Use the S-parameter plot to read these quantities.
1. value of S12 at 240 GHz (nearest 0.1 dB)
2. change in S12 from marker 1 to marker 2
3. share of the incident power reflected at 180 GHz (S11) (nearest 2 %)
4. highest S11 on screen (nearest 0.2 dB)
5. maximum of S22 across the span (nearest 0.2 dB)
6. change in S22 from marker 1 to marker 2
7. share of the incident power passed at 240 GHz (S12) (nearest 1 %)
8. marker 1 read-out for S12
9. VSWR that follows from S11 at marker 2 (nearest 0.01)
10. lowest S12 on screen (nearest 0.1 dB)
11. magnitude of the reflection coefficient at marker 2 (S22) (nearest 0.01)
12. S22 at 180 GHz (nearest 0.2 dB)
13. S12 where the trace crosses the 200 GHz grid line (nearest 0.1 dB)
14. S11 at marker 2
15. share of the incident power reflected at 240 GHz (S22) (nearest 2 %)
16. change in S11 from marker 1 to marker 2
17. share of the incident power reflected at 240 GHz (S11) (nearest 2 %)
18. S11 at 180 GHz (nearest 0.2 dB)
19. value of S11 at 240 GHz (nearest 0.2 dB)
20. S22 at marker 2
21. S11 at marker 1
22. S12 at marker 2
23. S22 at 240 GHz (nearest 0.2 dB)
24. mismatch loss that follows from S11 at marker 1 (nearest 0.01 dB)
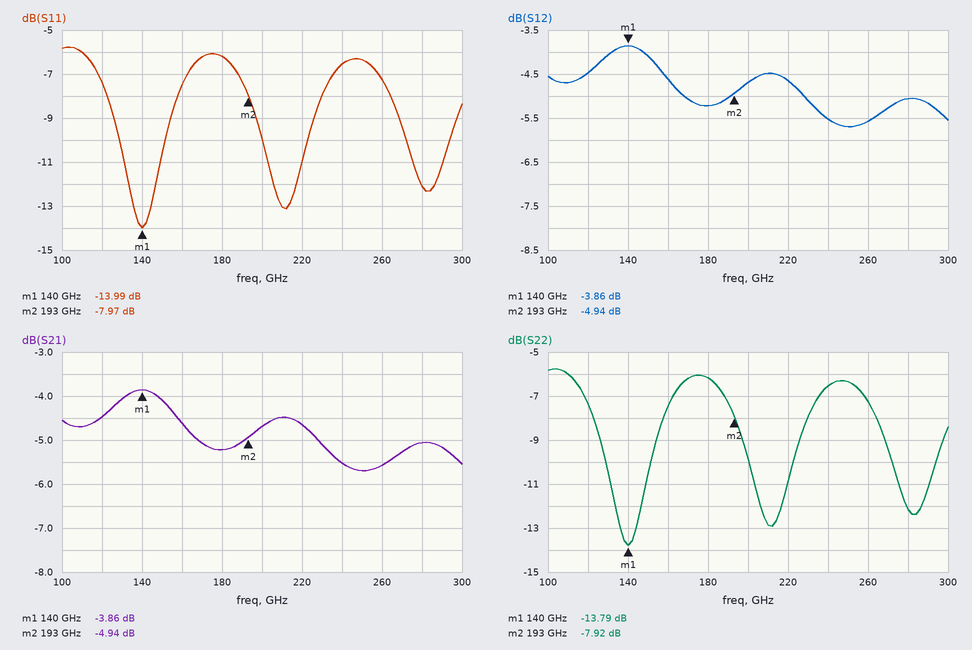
-5.5 dB
-1.08 dB
24 %
-5.8 dB
-5.8 dB
5.87 dB
28 %
-3.86 dB
2.33
-5.7 dB
0.40
-6.2 dB
-4.7 dB
-7.97 dB
22 %
6.02 dB
22 %
-6.2 dB
-6.6 dB
-7.92 dB
-13.99 dB
-4.94 dB
-6.6 dB
0.18 dB
